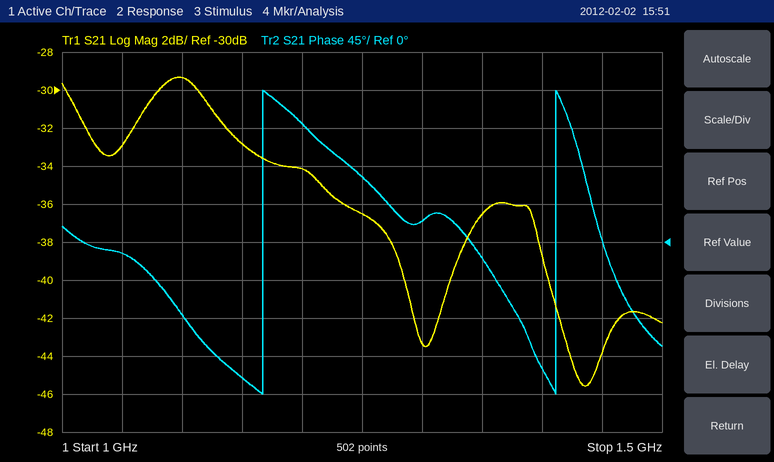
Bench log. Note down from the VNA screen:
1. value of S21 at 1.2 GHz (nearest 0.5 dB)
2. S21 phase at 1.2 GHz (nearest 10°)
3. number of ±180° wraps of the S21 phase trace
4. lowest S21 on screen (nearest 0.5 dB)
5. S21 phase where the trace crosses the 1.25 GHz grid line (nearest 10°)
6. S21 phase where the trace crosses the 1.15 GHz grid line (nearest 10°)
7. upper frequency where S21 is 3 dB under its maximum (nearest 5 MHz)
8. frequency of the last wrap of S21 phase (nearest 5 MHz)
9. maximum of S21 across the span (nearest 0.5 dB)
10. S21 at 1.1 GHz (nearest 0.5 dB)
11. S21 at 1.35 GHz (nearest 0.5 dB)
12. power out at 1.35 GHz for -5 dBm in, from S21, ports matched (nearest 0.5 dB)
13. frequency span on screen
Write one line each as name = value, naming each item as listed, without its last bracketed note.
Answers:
value of S21 at 1.2 GHz = -34.0 dB
S21 phase at 1.2 GHz = 140°
number of ±180° wraps of the S21 phase trace = 2
lowest S21 on screen = -45.5 dB
S21 phase where the trace crosses the 1.25 GHz grid line = 80°
S21 phase where the trace crosses the 1.15 GHz grid line = -160°
upper frequency where S21 is 3 dB under its maximum = 1.140 GHz
frequency of the last wrap of S21 phase = 1.410 GHz
maximum of S21 across the span = -29.5 dB
S21 at 1.1 GHz = -29.5 dB
S21 at 1.35 GHz = -36.5 dB
power out at 1.35 GHz for -5 dBm in, from S21, ports matched = -41.5 dBm
frequency span on screen = 500 MHz
